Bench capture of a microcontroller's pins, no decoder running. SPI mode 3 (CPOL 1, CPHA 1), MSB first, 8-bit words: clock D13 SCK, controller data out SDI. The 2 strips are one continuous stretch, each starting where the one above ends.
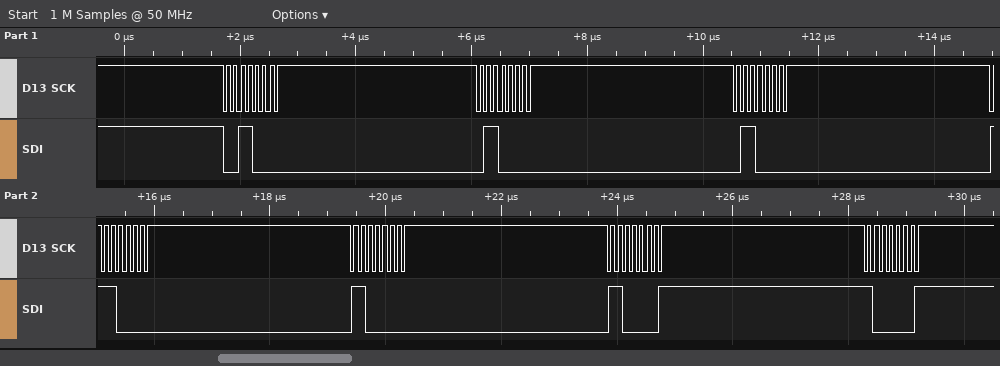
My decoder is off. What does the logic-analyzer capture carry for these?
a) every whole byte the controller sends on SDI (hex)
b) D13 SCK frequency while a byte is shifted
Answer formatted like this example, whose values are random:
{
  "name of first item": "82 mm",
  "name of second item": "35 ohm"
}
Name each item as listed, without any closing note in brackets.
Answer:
{
  "every whole byte the controller sends on SDI": "30 60 60 E0 C0 C1 81",
  "D13 SCK frequency while a byte is shifted": "8 MHz"
}
